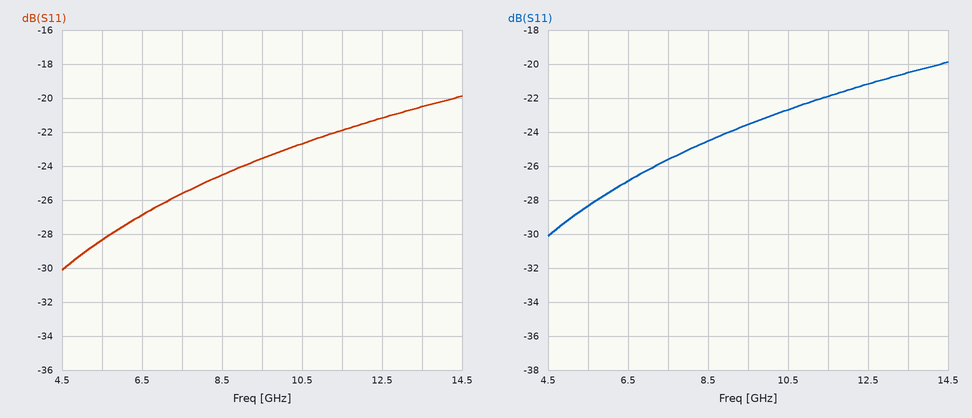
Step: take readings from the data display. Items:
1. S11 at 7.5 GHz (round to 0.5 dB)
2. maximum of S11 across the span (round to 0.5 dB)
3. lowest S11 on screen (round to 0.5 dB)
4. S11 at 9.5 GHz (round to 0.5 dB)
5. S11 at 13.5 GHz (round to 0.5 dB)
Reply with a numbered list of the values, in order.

1. -25.5 dB
2. -20.0 dB
3. -30.0 dB
4. -23.5 dB
5. -20.5 dB
